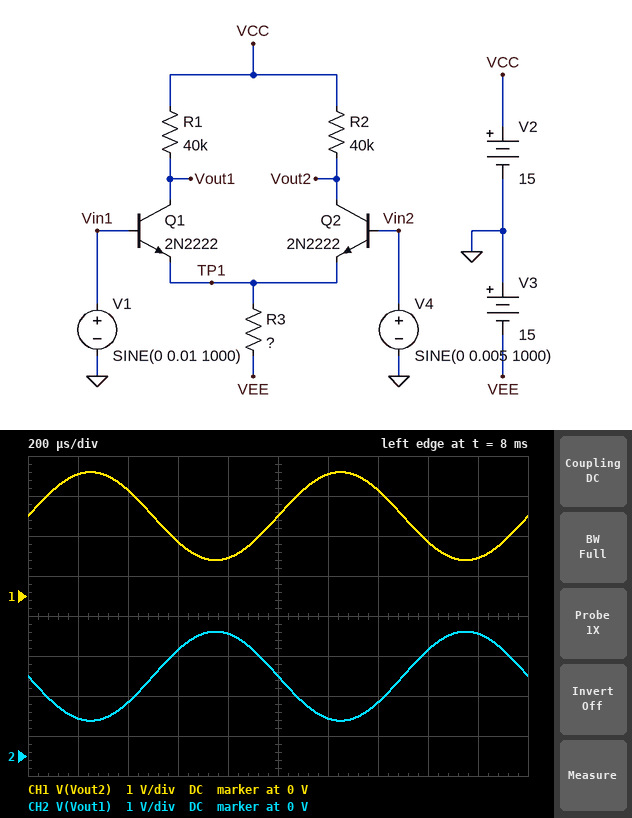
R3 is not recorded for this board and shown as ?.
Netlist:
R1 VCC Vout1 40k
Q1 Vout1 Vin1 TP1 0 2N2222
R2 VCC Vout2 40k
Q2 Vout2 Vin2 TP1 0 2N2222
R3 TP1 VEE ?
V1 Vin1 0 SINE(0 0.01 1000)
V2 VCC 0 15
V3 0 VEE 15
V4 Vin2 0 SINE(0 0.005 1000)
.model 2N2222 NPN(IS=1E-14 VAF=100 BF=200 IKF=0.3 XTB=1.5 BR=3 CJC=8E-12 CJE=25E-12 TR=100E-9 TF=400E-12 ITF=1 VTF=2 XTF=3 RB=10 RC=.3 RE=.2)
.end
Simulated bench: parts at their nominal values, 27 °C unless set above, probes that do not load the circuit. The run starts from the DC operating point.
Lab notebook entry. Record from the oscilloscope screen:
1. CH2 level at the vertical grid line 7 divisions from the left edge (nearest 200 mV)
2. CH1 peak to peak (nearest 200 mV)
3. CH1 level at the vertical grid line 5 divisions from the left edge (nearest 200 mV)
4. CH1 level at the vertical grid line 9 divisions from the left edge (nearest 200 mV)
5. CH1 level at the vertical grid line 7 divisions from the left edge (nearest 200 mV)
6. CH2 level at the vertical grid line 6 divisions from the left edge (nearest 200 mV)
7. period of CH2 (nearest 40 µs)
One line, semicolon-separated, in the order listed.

1.4 V; 2.2 V; 2.0 V; 1.0 V; 2.6 V; 1.0 V; 1.00 ms
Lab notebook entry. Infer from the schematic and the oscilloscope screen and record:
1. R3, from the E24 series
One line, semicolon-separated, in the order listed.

22 kΩ
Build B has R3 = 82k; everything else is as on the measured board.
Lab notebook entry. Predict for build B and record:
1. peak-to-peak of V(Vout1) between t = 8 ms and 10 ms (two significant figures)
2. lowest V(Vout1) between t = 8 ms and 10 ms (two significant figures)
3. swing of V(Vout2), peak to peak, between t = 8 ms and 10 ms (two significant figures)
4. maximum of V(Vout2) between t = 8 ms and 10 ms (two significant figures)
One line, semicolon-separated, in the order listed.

660 mV; 11 V; 650 mV; 12 V
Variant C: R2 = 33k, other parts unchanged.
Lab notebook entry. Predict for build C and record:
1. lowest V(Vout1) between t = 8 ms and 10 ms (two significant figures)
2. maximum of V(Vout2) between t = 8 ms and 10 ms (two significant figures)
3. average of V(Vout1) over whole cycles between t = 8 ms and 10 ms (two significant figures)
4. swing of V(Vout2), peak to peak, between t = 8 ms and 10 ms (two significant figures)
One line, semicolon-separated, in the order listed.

1.0 V; 5.1 V; 2.1 V; 1.8 V
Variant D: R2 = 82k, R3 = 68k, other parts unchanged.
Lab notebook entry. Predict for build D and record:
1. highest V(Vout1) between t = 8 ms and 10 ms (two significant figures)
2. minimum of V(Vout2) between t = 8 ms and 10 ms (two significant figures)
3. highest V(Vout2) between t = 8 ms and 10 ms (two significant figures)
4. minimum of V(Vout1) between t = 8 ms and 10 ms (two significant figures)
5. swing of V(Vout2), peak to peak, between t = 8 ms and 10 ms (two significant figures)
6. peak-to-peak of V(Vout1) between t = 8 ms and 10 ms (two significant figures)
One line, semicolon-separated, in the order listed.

11 V; 5.7 V; 7.3 V; 10 V; 1.6 V; 770 mV
